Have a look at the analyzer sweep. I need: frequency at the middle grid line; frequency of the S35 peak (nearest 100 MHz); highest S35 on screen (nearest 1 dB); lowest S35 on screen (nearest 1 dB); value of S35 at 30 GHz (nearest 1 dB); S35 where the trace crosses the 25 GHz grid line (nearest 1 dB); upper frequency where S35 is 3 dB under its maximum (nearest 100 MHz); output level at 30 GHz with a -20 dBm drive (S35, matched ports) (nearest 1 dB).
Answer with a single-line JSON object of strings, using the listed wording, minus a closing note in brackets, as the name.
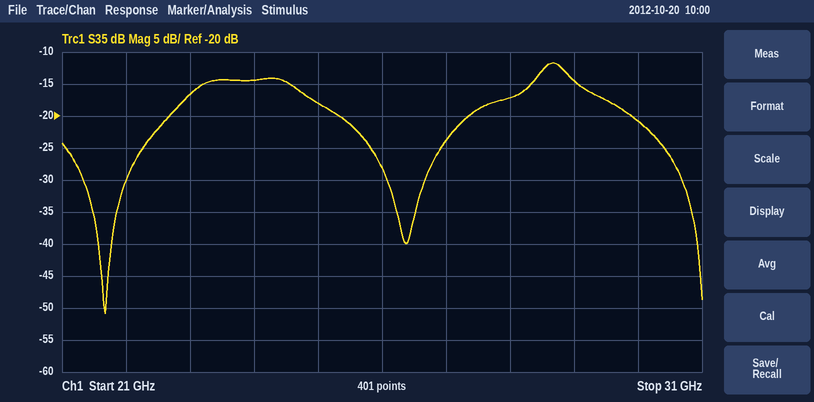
{"frequency at the middle grid line": "26 GHz", "frequency of the S35 peak": "28.7 GHz", "highest S35 on screen": "-12 dB", "lowest S35 on screen": "-51 dB", "value of S35 at 30 GHz": "-21 dB", "S35 where the trace crosses the 25 GHz grid line": "-18 dB", "upper frequency where S35 is 3 dB under its maximum": "29.0 GHz", "output level at 30 GHz with a -20 dBm drive (S35, matched ports)": "-41 dBm"}
